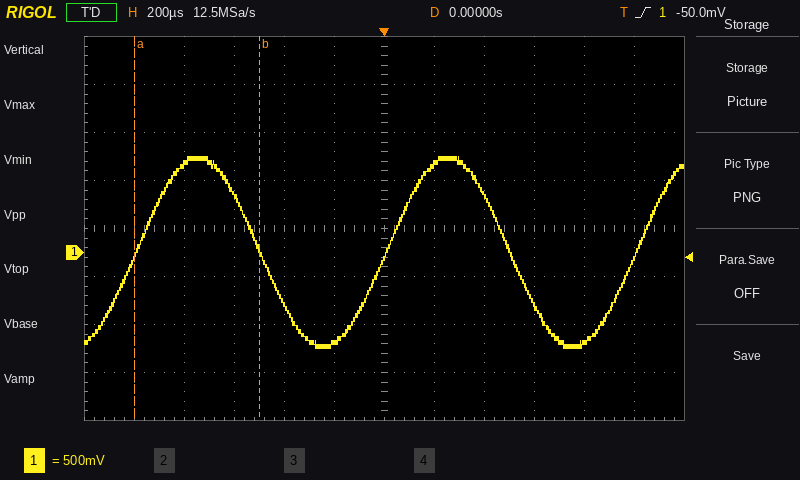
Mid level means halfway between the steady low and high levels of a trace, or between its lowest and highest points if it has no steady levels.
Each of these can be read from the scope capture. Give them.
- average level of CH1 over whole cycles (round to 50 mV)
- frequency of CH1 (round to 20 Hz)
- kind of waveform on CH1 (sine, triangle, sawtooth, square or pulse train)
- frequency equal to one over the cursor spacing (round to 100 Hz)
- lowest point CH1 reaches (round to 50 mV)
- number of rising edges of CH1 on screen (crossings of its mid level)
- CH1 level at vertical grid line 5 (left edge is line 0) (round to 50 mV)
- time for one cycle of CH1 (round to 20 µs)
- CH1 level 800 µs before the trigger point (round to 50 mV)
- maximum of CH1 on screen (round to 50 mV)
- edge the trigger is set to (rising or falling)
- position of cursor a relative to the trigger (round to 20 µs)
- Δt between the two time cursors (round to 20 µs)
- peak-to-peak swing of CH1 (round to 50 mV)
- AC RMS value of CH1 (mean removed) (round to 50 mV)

0 mV
1.00 kHz
sine
2.0 kHz
-1.00 V
3
-950 mV
1.00 ms
900 mV
1.00 V
rising
-1.00 ms
500 µs
2.00 V
700 mV
